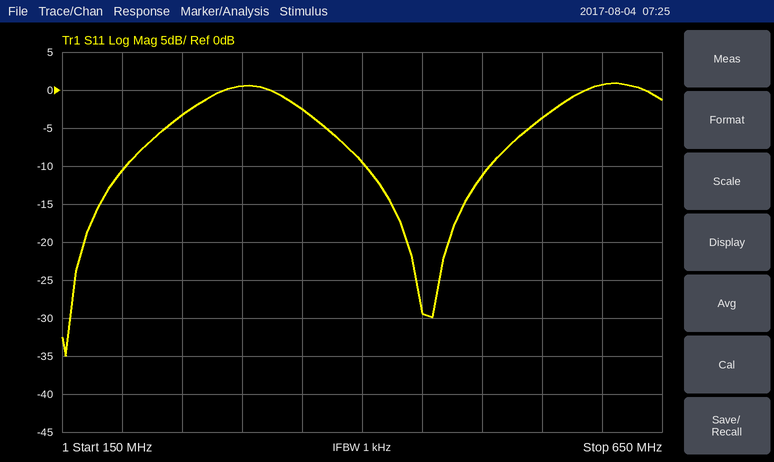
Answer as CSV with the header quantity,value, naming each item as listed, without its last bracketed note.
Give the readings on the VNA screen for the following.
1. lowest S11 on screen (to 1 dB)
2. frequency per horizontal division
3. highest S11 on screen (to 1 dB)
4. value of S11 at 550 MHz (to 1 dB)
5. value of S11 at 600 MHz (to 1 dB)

quantity,value
lowest S11 on screen,-35 dB
frequency per horizontal division,50 MHz
highest S11 on screen,1 dB
value of S11 at 550 MHz,-4 dB
value of S11 at 600 MHz,1 dB
